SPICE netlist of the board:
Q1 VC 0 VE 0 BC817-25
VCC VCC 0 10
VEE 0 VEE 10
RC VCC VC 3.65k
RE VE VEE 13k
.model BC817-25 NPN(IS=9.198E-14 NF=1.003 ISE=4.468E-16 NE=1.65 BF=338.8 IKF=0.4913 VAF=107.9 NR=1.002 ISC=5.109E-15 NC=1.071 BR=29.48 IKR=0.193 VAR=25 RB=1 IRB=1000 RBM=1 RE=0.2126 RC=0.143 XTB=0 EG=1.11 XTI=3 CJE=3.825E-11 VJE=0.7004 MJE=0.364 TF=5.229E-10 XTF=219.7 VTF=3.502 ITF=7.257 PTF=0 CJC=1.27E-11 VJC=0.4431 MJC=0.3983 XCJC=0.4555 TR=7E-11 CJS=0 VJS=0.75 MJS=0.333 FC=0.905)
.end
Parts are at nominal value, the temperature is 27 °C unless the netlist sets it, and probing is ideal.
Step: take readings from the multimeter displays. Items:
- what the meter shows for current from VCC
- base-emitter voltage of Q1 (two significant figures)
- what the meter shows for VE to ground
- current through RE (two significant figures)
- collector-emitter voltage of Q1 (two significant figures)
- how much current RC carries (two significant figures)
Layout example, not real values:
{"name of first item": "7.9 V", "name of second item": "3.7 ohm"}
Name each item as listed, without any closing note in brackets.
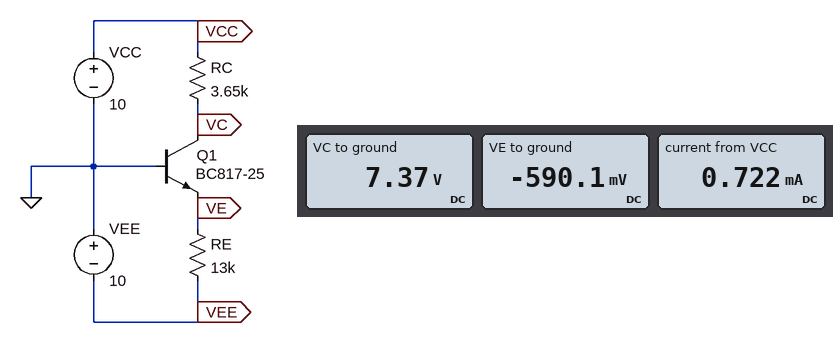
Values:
{"what the meter shows for current from VCC": "0.722 mA", "base-emitter voltage of Q1": "590 mV", "what the meter shows for VE to ground": "-590.1 mV", "current through RE": "720 µA", "collector-emitter voltage of Q1": "8.0 V", "how much current RC carries": "720 µA"}
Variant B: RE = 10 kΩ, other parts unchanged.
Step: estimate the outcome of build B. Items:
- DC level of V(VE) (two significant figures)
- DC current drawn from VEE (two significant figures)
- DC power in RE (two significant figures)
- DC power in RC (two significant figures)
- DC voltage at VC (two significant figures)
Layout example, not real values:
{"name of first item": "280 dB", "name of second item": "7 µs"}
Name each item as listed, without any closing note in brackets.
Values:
{"DC level of V(VE)": "-600 mV", "DC current drawn from VEE": "940 µA", "DC power in RE": "8.8 mW", "DC power in RC": "3.2 mW", "DC voltage at VC": "6.6 V"}
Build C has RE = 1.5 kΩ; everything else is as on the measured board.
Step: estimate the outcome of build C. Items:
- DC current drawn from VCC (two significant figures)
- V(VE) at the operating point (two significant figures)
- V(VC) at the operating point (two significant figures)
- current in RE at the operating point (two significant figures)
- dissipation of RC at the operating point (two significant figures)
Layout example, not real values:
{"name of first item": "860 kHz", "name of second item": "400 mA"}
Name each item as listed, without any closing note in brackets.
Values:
{"DC current drawn from VCC": "2.9 mA", "V(VE) at the operating point": "-720 mV", "V(VC) at the operating point": "-710 mV", "current in RE at the operating point": "6.2 mA", "dissipation of RC at the operating point": "31 mW"}
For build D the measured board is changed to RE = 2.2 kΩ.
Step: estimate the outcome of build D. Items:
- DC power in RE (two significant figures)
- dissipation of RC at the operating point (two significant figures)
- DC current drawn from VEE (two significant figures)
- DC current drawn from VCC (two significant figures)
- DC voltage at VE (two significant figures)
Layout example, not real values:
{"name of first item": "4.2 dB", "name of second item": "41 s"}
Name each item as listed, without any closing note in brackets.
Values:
{"DC power in RE": "39 mW", "dissipation of RC at the operating point": "31 mW", "DC current drawn from VEE": "4.2 mA", "DC current drawn from VCC": "2.9 mA", "DC voltage at VE": "-690 mV"}
